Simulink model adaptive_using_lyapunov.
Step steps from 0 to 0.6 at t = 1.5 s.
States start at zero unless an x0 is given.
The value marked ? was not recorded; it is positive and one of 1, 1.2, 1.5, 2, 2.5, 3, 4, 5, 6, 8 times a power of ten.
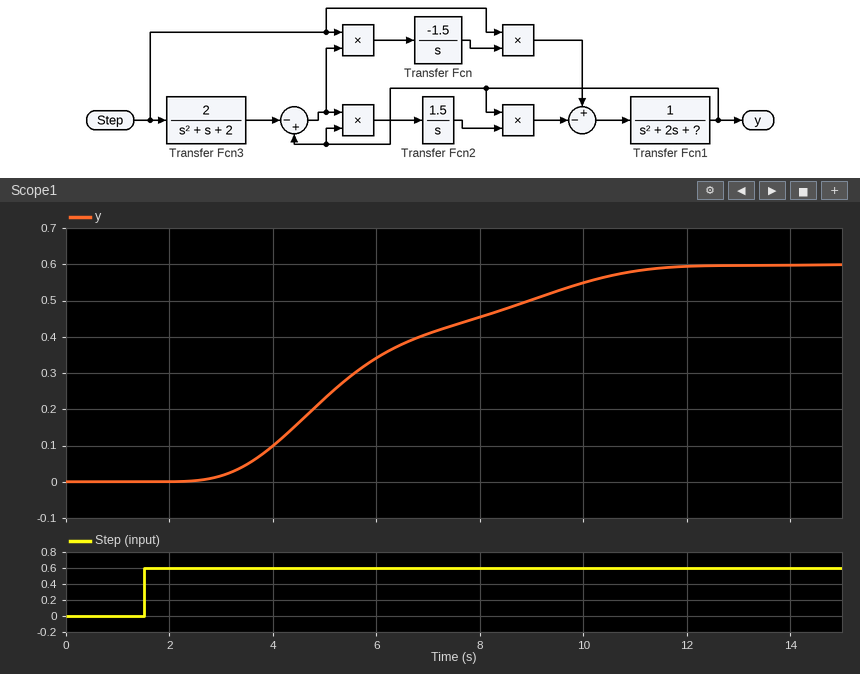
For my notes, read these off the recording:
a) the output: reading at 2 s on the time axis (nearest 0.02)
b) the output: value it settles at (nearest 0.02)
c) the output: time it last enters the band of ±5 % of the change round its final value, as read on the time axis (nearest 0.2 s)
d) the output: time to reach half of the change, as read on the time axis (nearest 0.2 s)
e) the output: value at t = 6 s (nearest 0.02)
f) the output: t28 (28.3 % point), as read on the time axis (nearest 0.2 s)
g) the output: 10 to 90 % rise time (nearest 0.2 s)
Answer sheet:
0.00
0.60
10.6 s
5.6 s
0.34
4.6 s
6.2 s
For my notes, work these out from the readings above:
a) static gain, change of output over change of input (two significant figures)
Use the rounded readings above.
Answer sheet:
1.0
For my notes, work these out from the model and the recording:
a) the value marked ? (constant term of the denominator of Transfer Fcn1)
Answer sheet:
3
